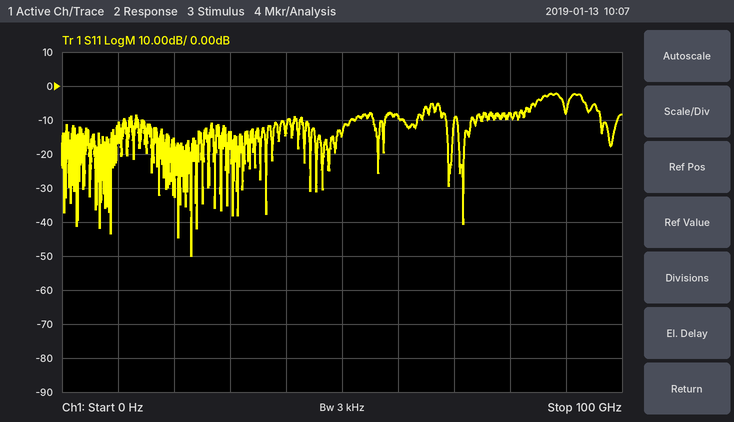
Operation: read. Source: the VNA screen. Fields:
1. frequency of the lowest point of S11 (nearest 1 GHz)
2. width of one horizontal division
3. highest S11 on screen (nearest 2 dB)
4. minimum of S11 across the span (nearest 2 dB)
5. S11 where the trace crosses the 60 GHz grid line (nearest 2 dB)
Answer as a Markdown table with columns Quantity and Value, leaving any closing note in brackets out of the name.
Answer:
| Quantity | Value |
|---|---|
| frequency of the lowest point of S11 | 23 GHz |
| width of one horizontal division | 10 GHz |
| highest S11 on screen | -2 dB |
| minimum of S11 across the span | -50 dB |
| S11 where the trace crosses the 60 GHz grid line | -8 dB |
